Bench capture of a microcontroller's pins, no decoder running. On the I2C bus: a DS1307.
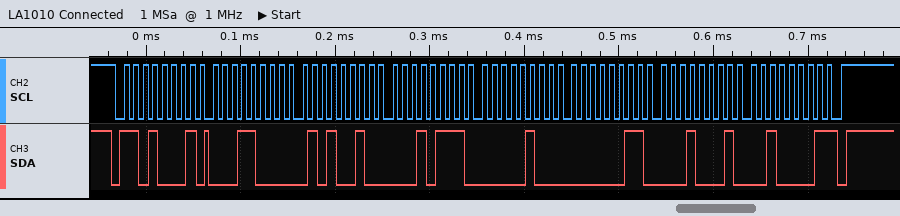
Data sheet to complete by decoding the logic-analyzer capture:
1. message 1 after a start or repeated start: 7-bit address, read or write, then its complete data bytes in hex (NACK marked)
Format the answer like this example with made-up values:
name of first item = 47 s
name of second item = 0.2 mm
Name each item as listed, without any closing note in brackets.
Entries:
message 1 after a start or repeated start: 7-bit address, read or write, then its complete data bytes in hex = 0x68 read: 18 52 17 04 03 11 21 NACK
